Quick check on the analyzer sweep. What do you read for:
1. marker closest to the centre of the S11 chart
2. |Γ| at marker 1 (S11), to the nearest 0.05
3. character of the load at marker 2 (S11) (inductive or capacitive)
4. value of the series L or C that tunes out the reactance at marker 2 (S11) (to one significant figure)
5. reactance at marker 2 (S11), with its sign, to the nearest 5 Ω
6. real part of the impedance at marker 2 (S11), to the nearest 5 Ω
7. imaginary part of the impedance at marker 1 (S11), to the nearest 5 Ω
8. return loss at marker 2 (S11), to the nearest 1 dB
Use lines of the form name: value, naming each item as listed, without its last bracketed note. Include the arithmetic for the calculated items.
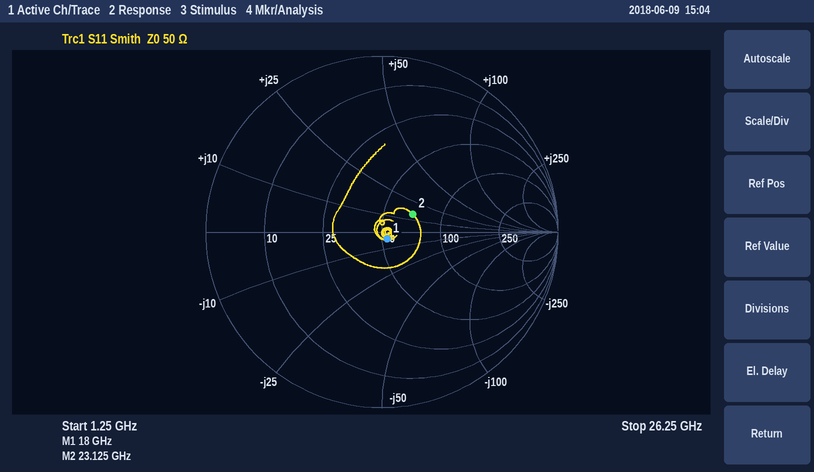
marker closest to the centre of the S11 chart: marker 1
|Γ| at marker 1 (S11), to the nearest 0.05: 0.05
character of the load at marker 2 (S11): inductive
value of the series L or C that tunes out the reactance at marker 2 (S11): C = 1/(2π × 23.125 GHz × 15 Ω) ≈ 459 fF, so 500 fF to one significant figure
reactance at marker 2 (S11), with its sign, to the nearest 5 Ω: +15 Ω
real part of the impedance at marker 2 (S11), to the nearest 5 Ω: 70 Ω
imaginary part of the impedance at marker 1 (S11), to the nearest 5 Ω: -5 Ω
return loss at marker 2 (S11), to the nearest 1 dB: 14 dB
